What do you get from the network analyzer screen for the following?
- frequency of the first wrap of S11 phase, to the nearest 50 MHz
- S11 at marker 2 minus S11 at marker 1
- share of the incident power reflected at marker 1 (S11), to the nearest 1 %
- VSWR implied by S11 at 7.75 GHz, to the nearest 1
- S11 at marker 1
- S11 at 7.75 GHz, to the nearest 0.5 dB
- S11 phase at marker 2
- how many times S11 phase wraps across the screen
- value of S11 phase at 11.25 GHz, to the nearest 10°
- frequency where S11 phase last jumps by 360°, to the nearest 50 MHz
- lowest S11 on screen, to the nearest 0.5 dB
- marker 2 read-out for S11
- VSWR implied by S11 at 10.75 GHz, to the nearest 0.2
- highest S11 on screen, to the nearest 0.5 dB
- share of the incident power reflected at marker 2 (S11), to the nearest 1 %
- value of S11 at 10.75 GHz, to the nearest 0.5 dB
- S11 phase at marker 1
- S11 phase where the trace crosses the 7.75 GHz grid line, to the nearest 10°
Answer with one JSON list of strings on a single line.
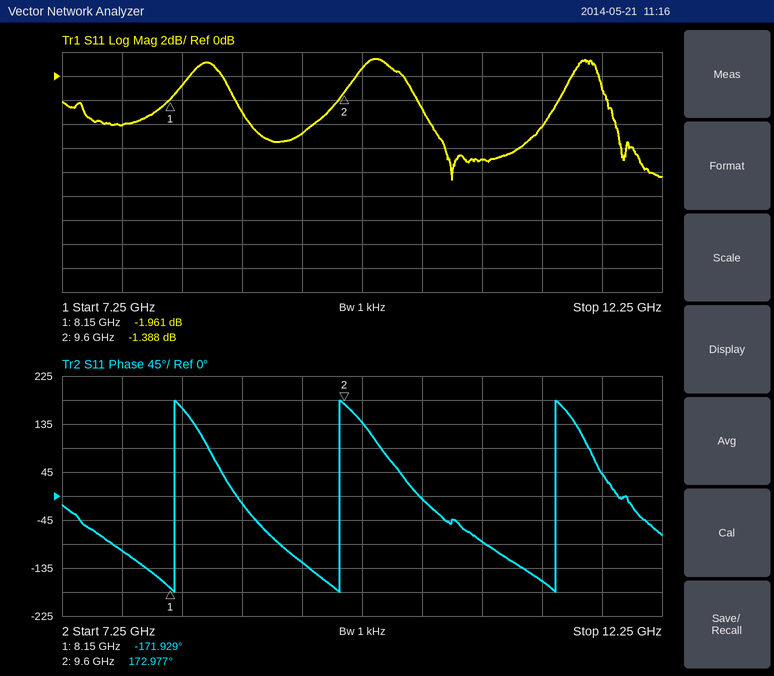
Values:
["8.20 GHz", "0.573 dB", "64 %", "4", "-1.961 dB", "-4.0 dB", "172.977°", "3", "-160°", "11.35 GHz", "-8.5 dB", "-1.388 dB", "2.6", "1.5 dB", "73 %", "-7.0 dB", "-171.929°", "-100°"]
